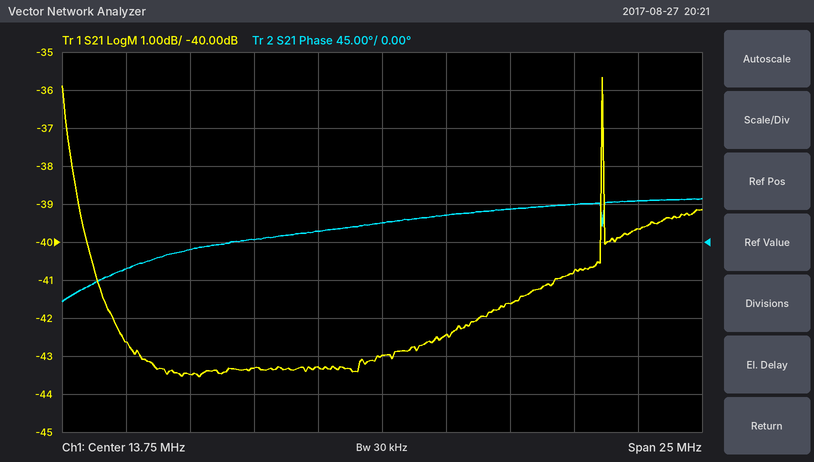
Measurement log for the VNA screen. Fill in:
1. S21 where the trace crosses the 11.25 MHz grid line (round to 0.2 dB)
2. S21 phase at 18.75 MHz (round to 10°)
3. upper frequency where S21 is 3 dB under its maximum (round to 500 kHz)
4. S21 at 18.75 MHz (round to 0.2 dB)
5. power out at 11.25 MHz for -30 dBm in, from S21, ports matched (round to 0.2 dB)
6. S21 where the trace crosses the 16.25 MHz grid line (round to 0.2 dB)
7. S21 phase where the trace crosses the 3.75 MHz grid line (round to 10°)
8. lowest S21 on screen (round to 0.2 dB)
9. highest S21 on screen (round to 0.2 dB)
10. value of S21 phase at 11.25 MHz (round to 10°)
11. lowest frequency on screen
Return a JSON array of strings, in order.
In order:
["-43.2 dB", "40°", "22.5 MHz", "-41.6 dB", "-73.2 dBm", "-42.4 dB", "-30°", "-43.6 dB", "-35.6 dB", "10°", "1.25 MHz"]
